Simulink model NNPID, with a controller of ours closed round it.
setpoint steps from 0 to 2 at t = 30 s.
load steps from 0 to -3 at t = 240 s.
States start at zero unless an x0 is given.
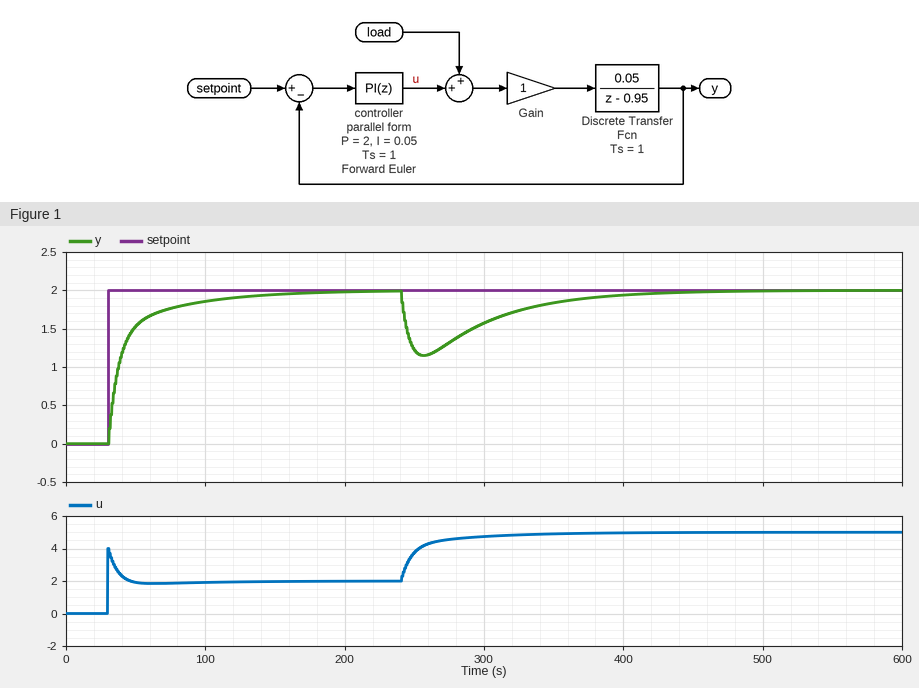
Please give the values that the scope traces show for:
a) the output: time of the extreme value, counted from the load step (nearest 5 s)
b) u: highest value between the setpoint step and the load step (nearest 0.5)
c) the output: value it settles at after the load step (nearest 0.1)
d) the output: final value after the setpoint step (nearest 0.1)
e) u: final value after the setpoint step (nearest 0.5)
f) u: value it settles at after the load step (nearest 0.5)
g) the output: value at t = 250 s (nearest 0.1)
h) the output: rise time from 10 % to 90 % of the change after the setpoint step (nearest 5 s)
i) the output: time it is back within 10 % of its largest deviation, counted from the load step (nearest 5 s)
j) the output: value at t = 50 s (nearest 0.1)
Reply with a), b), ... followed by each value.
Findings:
a) 15 s
b) 4.0
c) 2.0
d) 2.0
e) 2.0
f) 5.0
g) 1.2
h) 50 s
i) 145 s
j) 1.5
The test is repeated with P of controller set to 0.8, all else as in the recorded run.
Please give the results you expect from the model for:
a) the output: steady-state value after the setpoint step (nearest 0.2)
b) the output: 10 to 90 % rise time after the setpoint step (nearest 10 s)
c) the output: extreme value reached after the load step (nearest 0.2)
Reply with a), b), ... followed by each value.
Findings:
a) 2.0
b) 40 s
c) 0.8
